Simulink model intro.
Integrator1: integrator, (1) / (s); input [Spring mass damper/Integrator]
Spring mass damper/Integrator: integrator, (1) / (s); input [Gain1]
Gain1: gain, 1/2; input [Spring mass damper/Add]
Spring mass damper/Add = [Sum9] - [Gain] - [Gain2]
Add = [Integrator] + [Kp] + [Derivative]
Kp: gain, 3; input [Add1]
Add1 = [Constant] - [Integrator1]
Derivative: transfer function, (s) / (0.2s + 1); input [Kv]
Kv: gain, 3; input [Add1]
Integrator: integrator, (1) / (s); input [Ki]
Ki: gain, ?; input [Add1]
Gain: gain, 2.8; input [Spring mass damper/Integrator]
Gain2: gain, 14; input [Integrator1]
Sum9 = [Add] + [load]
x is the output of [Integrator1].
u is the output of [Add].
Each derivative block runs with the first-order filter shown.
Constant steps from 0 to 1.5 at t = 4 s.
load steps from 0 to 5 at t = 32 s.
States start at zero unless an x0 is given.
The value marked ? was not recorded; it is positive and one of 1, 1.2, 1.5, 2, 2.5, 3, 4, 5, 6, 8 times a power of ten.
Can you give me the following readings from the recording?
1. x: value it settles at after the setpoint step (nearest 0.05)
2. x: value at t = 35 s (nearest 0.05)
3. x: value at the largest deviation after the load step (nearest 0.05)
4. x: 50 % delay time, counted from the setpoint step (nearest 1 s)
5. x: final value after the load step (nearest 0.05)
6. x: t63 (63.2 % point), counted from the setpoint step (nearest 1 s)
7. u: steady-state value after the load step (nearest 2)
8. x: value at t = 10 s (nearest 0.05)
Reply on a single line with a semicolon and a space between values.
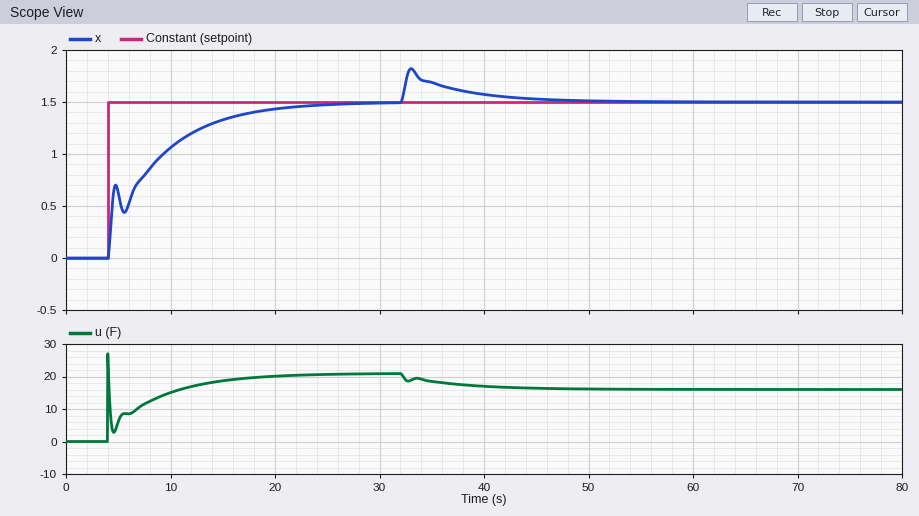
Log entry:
1.50; 1.70; 1.80; 3 s; 1.50; 5 s; 16; 1.05
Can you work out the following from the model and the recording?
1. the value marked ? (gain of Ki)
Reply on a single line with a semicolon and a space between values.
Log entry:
3
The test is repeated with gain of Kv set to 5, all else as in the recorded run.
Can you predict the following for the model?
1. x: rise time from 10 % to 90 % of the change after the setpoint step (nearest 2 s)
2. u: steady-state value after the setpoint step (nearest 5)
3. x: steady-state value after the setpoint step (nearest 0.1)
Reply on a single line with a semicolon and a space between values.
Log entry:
12 s; 20; 1.5
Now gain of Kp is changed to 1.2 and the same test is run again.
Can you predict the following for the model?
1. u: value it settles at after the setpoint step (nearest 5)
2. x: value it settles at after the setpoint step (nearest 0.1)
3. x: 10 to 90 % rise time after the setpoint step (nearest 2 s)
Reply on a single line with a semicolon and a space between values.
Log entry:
20; 1.5; 10 s
